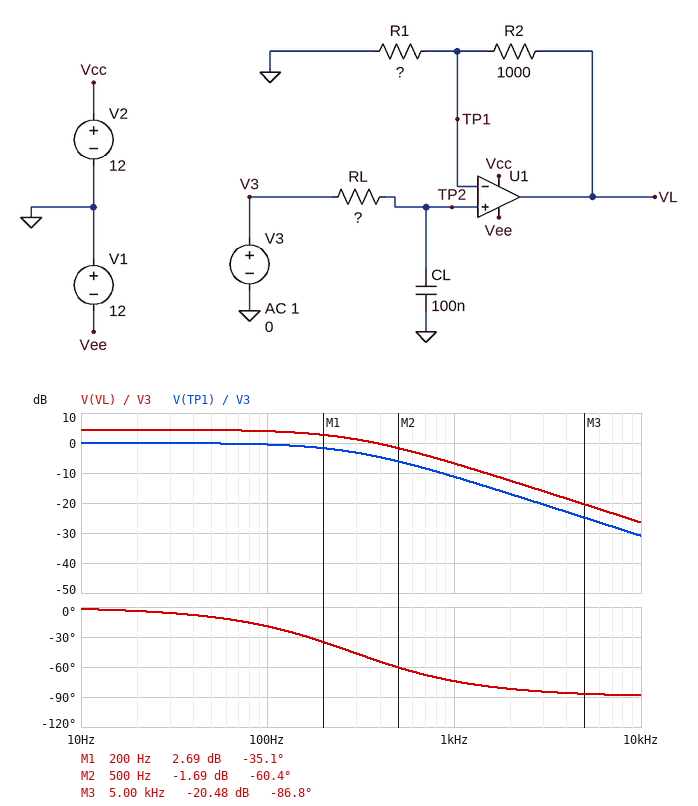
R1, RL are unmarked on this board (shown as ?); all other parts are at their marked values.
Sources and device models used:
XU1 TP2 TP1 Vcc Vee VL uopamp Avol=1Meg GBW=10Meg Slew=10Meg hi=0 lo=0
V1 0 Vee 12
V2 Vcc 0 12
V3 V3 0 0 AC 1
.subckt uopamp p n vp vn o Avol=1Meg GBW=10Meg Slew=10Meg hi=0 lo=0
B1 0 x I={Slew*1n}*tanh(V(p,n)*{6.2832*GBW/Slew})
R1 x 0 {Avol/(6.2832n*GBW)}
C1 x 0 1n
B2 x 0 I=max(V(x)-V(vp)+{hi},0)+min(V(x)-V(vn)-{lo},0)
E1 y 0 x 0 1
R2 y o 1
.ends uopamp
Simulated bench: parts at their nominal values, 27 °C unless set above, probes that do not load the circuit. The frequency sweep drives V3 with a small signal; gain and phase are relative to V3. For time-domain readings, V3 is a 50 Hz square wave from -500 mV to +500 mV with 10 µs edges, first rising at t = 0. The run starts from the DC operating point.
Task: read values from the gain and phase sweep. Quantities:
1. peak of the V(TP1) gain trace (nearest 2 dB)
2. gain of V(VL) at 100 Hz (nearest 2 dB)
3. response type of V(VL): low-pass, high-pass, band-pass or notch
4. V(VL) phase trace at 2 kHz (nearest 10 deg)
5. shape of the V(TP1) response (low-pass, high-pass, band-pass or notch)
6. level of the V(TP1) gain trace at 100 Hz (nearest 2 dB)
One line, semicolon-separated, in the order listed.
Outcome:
0 dB; 4 dB; low-pass; -80 deg; low-pass; 0 dB
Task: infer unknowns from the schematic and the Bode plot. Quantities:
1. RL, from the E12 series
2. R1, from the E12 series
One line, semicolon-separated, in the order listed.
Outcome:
5.6 kΩ; 1.5 kΩ
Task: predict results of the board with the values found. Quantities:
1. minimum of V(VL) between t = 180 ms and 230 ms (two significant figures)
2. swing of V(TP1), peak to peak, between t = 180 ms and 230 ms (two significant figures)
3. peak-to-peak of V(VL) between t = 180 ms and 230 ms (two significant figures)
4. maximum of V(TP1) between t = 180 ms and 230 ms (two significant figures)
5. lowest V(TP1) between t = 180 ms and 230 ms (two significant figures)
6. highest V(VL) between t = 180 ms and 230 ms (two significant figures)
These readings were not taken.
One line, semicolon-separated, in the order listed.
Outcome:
-830 mV; 1.0 V; 1.7 V; 500 mV; -500 mV; 830 mV
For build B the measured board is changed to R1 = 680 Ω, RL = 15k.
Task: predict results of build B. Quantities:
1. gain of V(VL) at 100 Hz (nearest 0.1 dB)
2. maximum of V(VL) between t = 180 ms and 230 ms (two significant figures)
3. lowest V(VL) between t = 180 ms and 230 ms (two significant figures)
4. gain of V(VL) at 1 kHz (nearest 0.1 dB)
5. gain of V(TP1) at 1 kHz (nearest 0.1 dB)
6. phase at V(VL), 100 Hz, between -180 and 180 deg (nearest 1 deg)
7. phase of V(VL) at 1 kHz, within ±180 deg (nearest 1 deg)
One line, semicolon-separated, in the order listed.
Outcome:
5.1 dB; 1.2 V; -1.2 V; -11.7 dB; -19.5 dB; -43 deg; -84 deg
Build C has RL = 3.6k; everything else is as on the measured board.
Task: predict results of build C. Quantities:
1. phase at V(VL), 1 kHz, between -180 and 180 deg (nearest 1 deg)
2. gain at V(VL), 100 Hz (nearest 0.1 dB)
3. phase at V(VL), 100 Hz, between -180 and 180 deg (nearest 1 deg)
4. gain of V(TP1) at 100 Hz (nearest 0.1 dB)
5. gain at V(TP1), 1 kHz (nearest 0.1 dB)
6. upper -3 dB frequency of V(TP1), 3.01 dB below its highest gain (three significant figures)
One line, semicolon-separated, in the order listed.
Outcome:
-66 deg; 4.2 dB; -13 deg; -0.2 dB; -7.9 dB; 442 Hz
